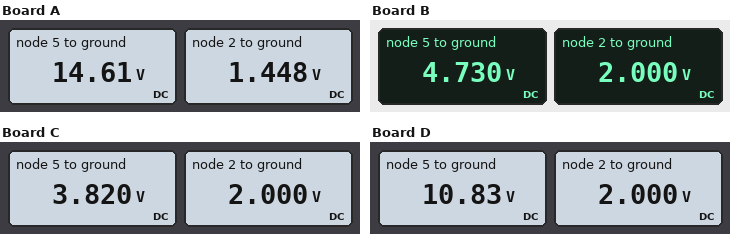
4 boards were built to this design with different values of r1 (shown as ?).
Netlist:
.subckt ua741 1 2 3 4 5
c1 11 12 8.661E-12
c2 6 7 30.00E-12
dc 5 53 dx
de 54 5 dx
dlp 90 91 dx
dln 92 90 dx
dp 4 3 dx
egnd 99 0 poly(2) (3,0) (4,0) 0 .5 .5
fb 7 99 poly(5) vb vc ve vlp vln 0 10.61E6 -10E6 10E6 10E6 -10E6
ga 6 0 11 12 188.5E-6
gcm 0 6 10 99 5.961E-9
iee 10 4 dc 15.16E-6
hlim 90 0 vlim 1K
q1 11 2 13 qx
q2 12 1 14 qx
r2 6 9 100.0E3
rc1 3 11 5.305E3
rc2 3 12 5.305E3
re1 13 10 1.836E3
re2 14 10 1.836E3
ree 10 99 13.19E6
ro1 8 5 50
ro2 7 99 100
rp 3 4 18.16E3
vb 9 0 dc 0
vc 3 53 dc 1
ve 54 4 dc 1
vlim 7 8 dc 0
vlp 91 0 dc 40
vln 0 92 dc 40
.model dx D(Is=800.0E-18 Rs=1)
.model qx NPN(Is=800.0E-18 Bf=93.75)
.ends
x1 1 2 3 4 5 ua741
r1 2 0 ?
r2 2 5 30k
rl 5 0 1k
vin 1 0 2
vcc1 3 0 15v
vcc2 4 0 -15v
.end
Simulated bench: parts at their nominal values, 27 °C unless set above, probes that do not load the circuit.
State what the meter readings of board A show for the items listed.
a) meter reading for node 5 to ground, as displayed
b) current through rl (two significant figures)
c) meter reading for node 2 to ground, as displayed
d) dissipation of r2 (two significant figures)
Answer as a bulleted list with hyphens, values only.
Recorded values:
- 14.61 V
- 15 mA
- 1.448 V
- 5.8 mW
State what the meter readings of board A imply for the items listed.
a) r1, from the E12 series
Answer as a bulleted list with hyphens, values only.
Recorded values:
- 3.3 kΩ
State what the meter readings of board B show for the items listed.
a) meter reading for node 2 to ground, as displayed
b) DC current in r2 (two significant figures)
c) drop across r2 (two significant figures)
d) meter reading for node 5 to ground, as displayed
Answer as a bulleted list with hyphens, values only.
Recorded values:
- 2.000 V
- 91 µA
- 2.7 V
- 4.730 V
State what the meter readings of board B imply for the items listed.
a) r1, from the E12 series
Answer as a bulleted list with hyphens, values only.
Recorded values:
- 22 kΩ
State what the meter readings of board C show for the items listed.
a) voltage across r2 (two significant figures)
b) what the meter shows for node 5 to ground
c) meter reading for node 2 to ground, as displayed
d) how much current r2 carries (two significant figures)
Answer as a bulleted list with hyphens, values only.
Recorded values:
- 1.8 V
- 3.820 V
- 2.000 V
- 61 µA
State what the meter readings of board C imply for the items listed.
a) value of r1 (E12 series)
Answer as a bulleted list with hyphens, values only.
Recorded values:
- 33 kΩ
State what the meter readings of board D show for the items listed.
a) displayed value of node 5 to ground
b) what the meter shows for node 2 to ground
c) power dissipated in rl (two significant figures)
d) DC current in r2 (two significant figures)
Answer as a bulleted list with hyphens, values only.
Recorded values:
- 10.83 V
- 2.000 V
- 120 mW
- 290 µA
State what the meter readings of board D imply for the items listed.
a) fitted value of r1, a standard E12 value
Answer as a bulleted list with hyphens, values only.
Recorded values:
- 6.8 kΩ
